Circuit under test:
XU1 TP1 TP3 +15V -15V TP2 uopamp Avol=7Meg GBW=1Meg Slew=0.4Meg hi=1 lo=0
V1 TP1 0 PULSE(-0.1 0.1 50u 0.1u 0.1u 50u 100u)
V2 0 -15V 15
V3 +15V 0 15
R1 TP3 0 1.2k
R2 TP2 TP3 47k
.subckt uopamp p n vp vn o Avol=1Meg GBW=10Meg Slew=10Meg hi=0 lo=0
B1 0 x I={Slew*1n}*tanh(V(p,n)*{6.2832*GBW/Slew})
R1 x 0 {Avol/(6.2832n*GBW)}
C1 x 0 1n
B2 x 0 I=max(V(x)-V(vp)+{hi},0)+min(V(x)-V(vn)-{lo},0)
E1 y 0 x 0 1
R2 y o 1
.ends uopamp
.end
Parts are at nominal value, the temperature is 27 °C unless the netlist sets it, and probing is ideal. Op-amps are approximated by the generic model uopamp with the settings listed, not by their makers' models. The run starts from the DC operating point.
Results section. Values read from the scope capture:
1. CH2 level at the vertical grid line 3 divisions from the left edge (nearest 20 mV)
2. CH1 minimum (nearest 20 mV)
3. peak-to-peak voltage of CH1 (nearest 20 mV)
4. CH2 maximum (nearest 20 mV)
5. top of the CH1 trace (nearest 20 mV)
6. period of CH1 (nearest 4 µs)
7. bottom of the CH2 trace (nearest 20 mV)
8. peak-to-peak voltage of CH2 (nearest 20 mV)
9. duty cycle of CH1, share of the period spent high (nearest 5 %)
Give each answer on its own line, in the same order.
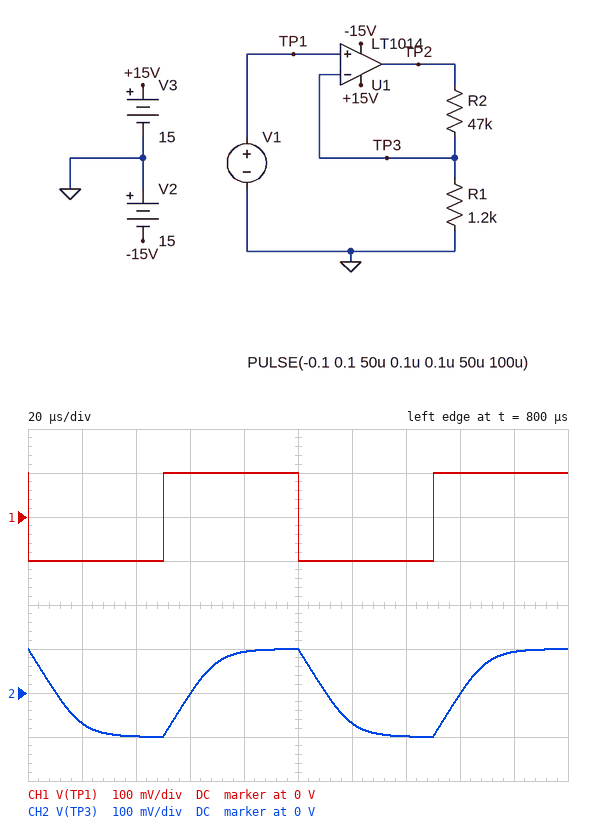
0 V
-100 mV
200 mV
100 mV
100 mV
100 µs
-100 mV
200 mV
50 %
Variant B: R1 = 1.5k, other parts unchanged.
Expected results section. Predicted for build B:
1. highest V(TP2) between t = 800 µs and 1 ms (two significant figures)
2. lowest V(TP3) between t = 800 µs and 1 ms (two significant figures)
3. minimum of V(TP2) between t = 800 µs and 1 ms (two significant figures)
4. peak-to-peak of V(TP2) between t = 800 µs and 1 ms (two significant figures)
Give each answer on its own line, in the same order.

3.2 V
-100 mV
-3.2 V
6.5 V
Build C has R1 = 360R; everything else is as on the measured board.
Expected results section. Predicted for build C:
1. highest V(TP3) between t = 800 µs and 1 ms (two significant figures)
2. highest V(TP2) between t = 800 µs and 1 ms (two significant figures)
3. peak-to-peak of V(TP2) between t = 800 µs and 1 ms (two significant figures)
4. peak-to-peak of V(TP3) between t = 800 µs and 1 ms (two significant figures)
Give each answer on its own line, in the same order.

64 mV
8.4 V
17 V
130 mV
